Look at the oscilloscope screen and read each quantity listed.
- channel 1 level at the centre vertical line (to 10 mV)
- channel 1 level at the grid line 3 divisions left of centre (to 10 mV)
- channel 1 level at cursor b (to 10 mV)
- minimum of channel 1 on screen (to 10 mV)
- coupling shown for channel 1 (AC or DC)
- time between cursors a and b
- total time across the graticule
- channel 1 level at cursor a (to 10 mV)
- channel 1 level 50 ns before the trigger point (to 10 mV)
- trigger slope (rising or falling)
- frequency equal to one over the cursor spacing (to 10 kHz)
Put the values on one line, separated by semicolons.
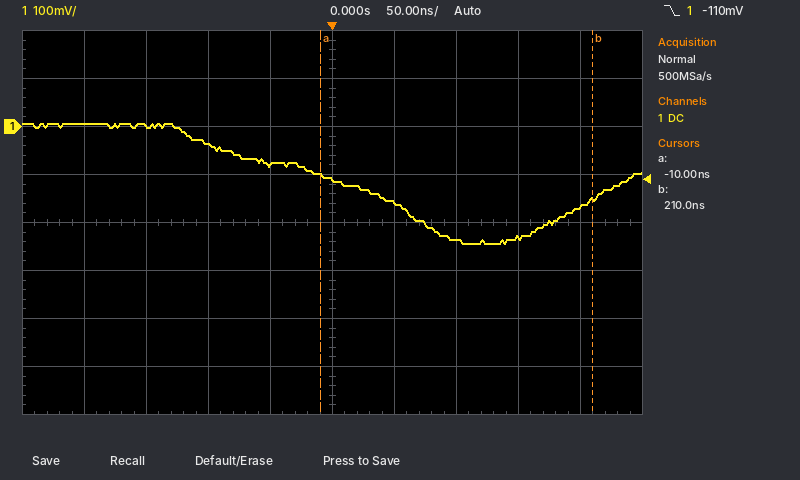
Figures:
-110 mV; 0 mV; -150 mV; -240 mV; DC; 220 ns; 500 ns; -100 mV; -80 mV; falling; 4.55 MHz
